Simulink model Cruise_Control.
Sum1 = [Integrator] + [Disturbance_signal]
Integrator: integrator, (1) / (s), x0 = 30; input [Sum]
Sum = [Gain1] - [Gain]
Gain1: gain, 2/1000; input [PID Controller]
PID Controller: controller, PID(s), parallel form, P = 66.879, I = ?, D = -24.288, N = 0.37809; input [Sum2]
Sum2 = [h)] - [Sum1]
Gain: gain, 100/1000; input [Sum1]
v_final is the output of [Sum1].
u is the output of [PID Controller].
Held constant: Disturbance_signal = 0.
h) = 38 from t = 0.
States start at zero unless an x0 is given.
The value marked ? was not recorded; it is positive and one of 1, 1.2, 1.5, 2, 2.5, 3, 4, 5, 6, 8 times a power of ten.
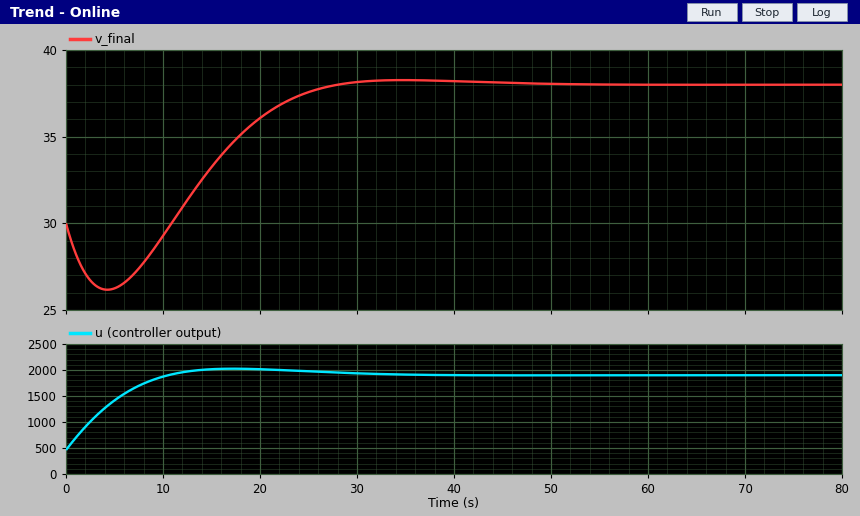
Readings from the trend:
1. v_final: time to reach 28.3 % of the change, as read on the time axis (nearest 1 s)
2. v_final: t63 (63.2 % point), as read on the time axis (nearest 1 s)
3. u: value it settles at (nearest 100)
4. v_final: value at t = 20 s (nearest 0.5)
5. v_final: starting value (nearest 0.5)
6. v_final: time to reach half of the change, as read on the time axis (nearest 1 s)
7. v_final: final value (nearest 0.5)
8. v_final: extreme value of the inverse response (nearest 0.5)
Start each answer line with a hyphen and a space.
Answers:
- 14 s
- 18 s
- 1900
- 36.0
- 30.0
- 16 s
- 38.0
- 26.0
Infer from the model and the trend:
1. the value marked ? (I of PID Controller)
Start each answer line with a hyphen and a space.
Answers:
- 12
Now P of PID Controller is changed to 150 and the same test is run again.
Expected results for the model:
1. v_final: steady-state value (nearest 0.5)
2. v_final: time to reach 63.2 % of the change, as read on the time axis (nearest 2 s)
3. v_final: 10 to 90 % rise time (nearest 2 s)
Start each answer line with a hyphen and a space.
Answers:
- 38.0
- 20 s
- 30 s
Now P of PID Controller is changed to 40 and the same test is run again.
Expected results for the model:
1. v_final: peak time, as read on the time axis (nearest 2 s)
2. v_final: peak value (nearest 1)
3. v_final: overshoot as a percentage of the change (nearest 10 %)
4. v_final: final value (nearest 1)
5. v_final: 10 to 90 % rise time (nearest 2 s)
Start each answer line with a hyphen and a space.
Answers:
- 30 s
- 39
- 20 %
- 38
- 8 s
